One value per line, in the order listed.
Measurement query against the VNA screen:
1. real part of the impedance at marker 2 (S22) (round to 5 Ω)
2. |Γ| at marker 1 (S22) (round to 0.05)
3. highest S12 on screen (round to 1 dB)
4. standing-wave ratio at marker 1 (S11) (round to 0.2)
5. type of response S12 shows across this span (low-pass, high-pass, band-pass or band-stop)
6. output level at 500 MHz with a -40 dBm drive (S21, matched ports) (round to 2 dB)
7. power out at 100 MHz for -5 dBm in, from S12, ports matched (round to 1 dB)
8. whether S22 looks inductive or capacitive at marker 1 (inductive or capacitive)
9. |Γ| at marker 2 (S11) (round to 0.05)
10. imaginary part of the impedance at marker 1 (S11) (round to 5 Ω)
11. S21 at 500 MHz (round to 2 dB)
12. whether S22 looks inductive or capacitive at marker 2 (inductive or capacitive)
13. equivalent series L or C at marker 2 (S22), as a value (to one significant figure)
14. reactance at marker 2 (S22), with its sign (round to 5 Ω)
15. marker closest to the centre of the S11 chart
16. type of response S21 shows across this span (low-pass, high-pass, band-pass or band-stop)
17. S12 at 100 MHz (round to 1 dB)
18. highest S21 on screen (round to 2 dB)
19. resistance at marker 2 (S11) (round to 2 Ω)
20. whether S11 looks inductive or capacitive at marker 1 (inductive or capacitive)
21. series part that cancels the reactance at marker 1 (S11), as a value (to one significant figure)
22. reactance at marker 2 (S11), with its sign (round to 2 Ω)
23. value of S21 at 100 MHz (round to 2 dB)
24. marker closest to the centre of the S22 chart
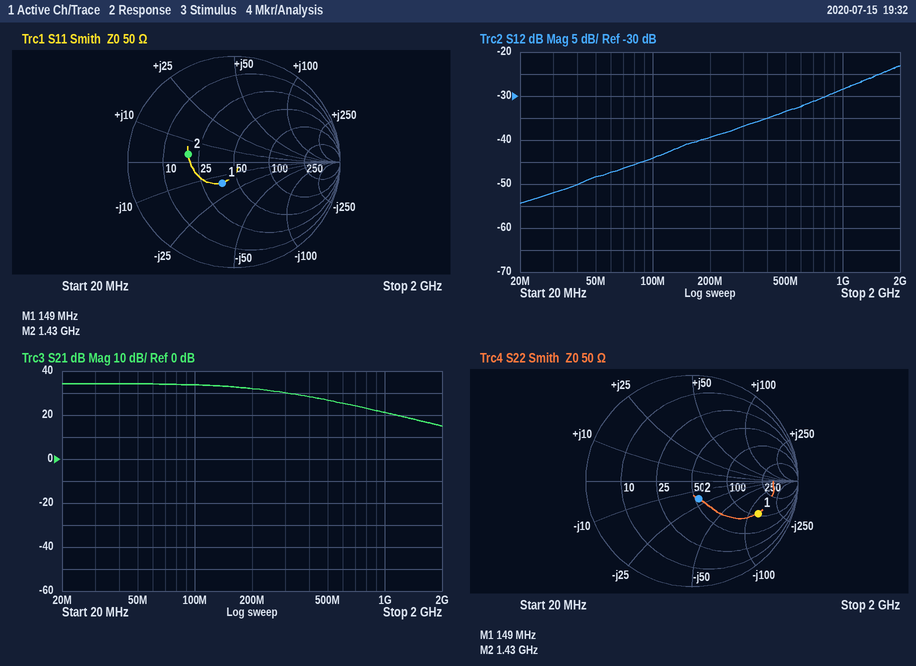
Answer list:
55 Ω
0.70
-23 dB
1.6
high-pass
-14 dBm
-49 dBm
capacitive
0.45
-15 Ω
26 dB
capacitive
6 pF
-20 Ω
marker 1
low-pass
-44 dB
34 dB
20 Ω
capacitive
20 nH
+4 Ω
34 dB
marker 2
